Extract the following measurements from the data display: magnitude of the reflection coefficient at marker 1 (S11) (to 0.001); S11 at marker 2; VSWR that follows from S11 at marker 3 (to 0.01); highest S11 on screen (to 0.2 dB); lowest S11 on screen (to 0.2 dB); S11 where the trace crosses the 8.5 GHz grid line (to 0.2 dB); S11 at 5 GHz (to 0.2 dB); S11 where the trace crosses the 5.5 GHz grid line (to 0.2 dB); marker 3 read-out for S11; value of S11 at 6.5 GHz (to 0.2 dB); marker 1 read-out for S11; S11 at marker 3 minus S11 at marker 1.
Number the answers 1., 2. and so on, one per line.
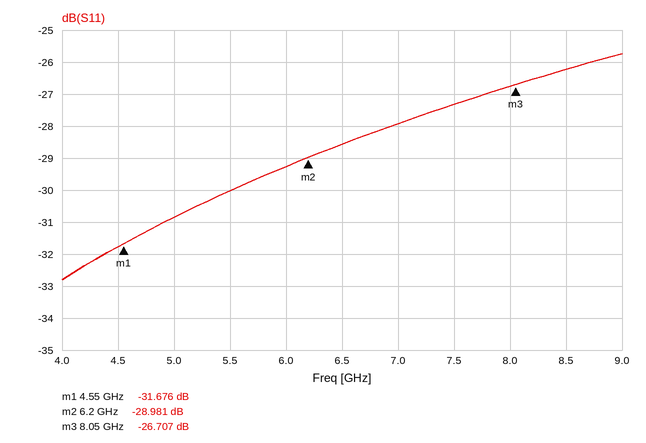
1. 0.026
2. -28.981 dB
3. 1.10
4. -25.8 dB
5. -32.8 dB
6. -26.2 dB
7. -30.8 dB
8. -30.0 dB
9. -26.707 dB
10. -28.6 dB
11. -31.676 dB
12. 4.969 dB
